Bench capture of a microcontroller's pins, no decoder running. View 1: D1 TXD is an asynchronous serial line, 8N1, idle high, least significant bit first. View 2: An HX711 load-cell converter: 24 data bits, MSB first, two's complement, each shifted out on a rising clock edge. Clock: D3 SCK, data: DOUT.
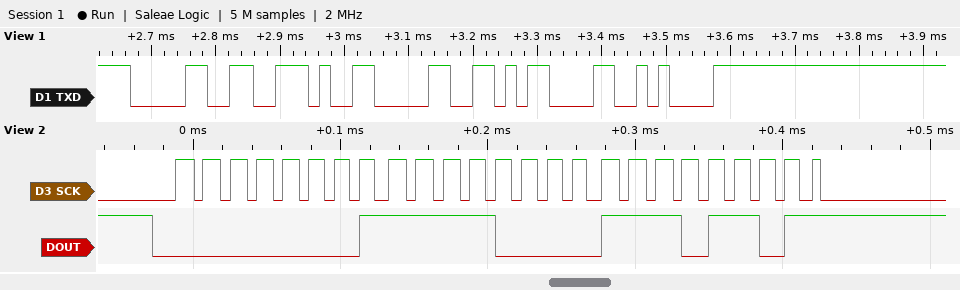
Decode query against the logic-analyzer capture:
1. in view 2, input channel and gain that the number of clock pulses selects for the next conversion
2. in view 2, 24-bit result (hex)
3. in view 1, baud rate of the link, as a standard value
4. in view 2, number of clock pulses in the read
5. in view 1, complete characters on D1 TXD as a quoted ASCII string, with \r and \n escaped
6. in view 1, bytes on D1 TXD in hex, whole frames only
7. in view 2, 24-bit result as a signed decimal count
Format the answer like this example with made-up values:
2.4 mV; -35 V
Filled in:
channel A, gain 128; 0x01F0ED; 57600 baud; 25; "0.0\r\n"; 30 2E 30 0D 0A; 127213
